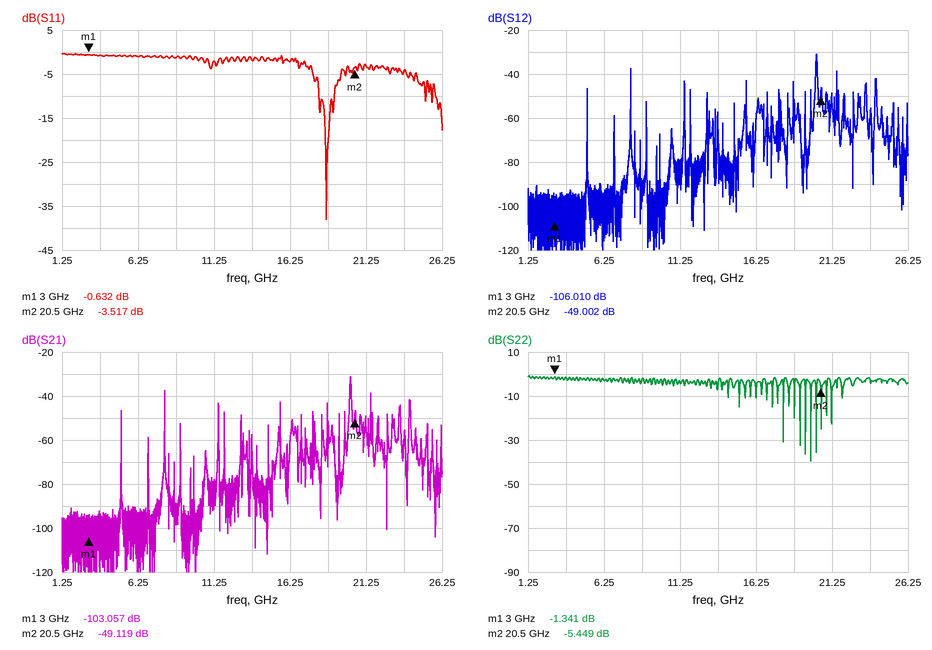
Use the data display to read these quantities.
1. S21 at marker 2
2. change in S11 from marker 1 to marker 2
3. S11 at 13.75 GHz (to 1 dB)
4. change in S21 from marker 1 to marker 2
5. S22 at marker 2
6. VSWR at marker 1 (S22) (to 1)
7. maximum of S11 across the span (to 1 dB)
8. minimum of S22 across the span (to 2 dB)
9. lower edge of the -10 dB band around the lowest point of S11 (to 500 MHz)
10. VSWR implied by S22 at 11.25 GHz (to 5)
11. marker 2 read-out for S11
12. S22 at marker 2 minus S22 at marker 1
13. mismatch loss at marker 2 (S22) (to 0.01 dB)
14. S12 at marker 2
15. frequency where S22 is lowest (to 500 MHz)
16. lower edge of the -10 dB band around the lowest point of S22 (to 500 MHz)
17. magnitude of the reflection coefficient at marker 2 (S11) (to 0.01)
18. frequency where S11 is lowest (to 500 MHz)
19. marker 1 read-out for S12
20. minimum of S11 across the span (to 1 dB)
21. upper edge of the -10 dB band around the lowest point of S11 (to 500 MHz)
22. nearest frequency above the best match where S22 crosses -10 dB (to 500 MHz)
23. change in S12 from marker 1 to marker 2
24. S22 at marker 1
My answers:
-49.119 dB
-2.885 dB
-2 dB
53.938 dB
-5.449 dB
13
0 dB
-40 dB
18.0 GHz
5
-3.517 dB
-4.108 dB
1.46 dB
-49.002 dB
20.0 GHz
20.0 GHz
0.67
18.5 GHz
-106.010 dB
-38 dB
19.0 GHz
20.0 GHz
57.008 dB
-1.341 dB
